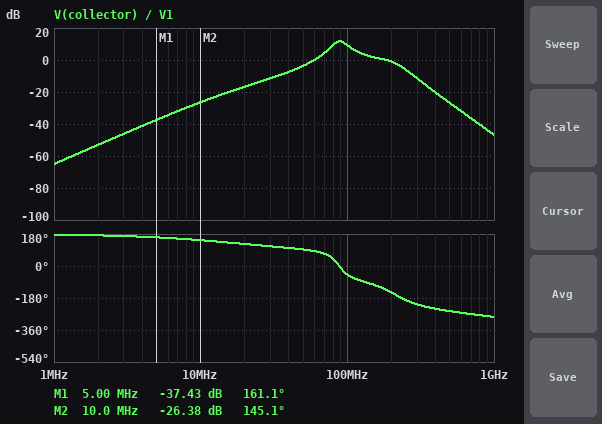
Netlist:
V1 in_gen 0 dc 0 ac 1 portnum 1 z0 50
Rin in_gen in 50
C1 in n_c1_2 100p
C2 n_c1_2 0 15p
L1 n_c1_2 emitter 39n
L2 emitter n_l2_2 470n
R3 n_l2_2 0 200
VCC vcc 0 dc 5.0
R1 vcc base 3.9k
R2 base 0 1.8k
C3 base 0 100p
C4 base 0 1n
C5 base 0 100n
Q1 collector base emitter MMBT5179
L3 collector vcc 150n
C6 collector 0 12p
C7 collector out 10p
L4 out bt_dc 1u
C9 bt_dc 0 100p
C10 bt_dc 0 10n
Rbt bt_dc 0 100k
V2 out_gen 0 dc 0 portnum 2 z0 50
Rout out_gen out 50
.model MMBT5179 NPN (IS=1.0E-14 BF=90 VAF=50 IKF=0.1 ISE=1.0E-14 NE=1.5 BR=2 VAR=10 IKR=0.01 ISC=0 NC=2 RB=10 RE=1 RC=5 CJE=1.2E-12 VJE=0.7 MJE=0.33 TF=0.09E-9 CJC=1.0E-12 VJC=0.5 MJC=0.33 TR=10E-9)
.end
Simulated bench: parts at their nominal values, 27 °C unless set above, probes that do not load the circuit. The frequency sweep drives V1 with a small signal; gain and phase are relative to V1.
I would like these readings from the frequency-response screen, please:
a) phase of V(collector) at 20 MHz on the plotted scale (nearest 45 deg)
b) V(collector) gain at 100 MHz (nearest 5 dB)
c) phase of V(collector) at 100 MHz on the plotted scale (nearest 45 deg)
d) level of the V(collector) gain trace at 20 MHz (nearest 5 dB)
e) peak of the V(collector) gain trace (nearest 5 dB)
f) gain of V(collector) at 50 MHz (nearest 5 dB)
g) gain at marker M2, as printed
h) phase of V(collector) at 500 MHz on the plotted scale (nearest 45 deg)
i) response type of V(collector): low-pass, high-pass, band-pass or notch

135 deg
10 dB
-45 deg
-15 dB
10 dB
-5 dB
-26.38 dB
-270 deg
band-pass
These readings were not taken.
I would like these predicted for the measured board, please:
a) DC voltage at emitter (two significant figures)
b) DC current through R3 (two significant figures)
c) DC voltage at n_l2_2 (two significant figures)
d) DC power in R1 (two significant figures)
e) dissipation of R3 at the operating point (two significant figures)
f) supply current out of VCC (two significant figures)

820 mV
4.1 mA
820 mV
3.1 mW
3.4 mW
5.0 mA
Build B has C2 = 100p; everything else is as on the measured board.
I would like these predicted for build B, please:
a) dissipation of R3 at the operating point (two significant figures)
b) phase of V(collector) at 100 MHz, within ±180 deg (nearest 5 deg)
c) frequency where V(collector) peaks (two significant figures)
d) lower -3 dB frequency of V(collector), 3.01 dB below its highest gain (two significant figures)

3.4 mW
-150 deg
85 MHz
75 MHz
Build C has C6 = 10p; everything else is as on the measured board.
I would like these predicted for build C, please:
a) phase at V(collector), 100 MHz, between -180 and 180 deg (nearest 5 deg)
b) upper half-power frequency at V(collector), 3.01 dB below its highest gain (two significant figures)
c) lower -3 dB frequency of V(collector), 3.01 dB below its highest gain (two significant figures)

-30 deg
110 MHz
81 MHz
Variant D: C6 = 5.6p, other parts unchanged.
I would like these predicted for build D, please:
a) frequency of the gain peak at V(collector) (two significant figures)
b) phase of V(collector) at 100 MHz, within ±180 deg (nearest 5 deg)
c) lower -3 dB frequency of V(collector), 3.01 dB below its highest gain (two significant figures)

110 MHz
15 deg
89 MHz
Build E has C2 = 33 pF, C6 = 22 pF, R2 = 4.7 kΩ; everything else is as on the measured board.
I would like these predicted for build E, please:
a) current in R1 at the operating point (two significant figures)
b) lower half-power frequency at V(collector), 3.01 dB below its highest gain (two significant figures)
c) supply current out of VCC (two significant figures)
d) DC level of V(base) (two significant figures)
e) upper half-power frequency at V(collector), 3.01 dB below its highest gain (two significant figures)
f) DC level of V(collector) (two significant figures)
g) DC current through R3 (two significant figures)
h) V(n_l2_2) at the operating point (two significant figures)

640 µA
68 MHz
9.4 mA
2.5 V
78 MHz
5.0 V
8.9 mA
1.8 V
